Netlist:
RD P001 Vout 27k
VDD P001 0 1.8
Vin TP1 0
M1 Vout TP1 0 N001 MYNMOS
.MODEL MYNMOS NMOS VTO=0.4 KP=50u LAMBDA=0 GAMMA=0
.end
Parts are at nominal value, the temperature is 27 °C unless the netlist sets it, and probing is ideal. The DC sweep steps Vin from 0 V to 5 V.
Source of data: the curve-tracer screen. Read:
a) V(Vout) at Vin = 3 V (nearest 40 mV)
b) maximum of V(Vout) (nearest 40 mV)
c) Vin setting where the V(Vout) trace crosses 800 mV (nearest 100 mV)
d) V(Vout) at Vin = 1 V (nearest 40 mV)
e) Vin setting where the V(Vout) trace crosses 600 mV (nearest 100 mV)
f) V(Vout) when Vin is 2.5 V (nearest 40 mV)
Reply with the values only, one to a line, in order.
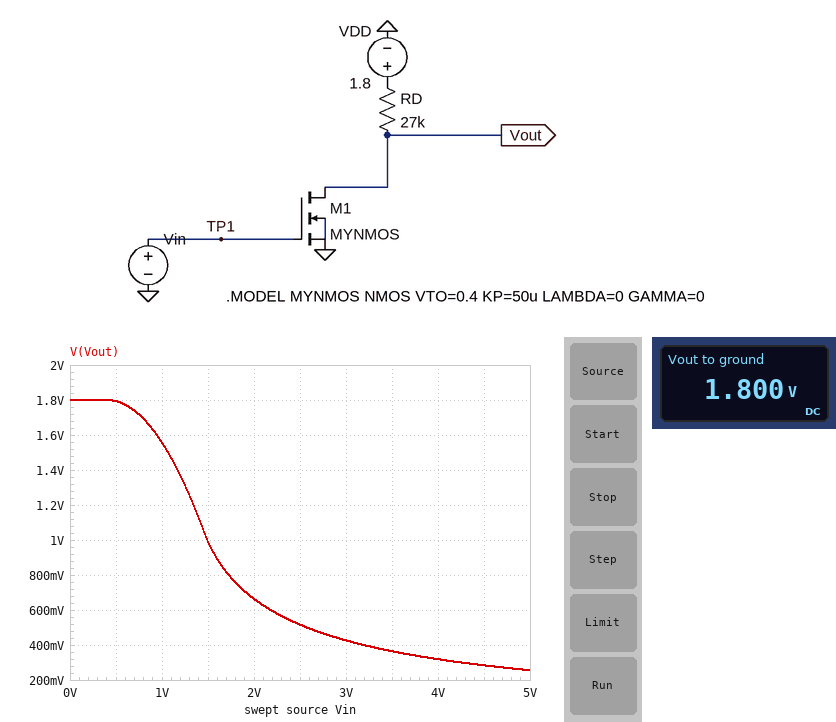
440 mV
1.80 V
1.7 V
1.56 V
2.2 V
520 mV
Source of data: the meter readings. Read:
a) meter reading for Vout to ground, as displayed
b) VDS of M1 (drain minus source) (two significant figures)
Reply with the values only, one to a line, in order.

1.800 V
1.8 V
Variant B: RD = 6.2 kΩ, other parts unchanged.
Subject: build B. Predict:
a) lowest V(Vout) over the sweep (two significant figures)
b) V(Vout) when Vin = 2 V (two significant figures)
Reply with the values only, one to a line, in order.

780 mV
1.4 V
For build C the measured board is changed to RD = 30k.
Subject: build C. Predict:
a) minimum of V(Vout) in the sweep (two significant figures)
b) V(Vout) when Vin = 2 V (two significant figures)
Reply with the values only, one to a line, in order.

230 mV
610 mV
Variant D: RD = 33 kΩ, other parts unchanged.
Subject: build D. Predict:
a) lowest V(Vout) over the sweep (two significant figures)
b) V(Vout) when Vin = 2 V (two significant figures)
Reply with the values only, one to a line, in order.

210 mV
570 mV
